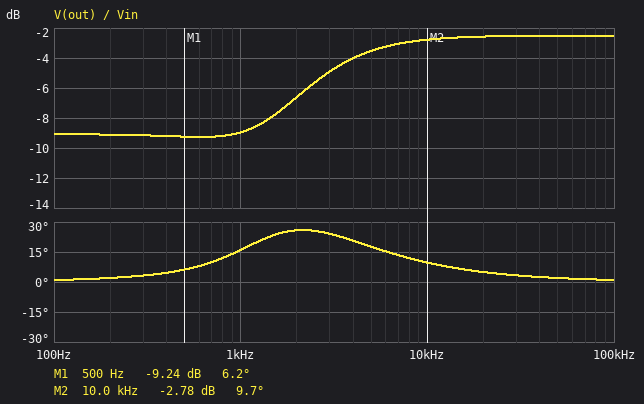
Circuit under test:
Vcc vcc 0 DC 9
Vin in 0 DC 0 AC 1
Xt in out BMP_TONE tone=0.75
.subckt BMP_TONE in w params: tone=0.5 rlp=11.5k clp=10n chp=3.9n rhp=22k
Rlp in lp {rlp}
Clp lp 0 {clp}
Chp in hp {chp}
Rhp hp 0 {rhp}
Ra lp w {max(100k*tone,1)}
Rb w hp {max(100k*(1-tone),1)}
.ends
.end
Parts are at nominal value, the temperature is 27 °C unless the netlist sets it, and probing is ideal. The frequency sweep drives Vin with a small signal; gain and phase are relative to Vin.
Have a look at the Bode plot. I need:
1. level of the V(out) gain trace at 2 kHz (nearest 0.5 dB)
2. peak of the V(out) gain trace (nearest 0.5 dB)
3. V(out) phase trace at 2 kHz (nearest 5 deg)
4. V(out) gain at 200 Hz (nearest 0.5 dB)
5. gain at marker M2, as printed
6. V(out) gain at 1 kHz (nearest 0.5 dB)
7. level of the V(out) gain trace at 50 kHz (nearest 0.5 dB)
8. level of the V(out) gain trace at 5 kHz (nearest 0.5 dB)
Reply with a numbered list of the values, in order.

1. -6.5 dB
2. -2.5 dB
3. 25 deg
4. -9.0 dB
5. -2.78 dB
6. -9.0 dB
7. -2.5 dB
8. -3.5 dB
